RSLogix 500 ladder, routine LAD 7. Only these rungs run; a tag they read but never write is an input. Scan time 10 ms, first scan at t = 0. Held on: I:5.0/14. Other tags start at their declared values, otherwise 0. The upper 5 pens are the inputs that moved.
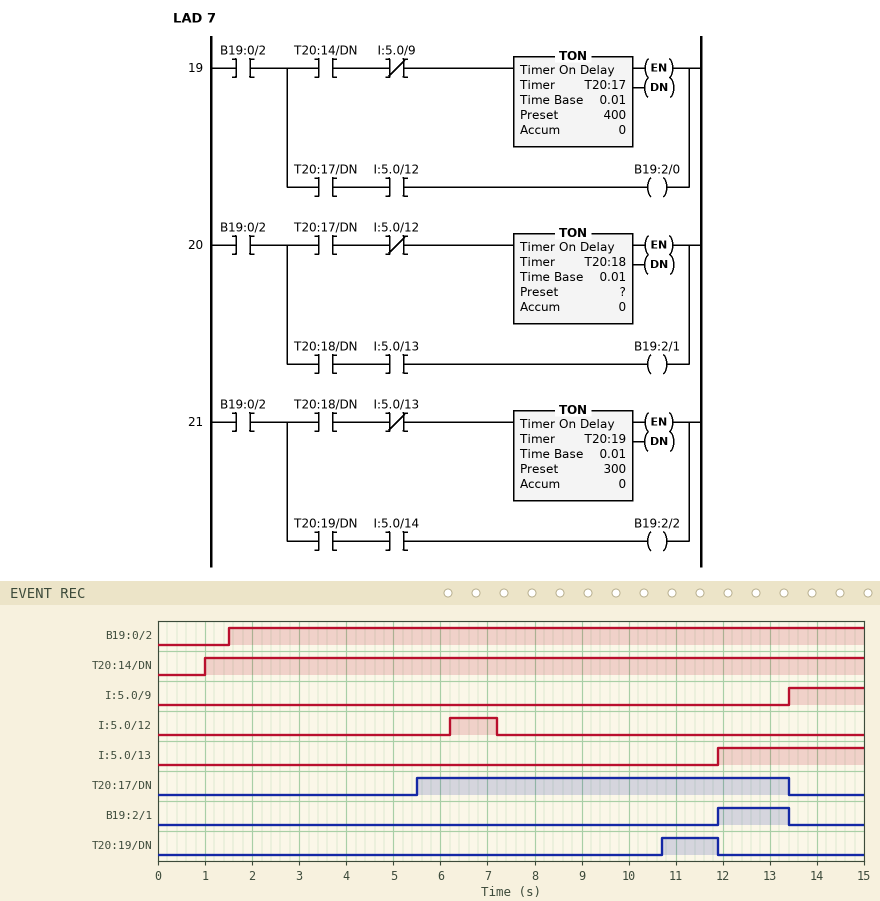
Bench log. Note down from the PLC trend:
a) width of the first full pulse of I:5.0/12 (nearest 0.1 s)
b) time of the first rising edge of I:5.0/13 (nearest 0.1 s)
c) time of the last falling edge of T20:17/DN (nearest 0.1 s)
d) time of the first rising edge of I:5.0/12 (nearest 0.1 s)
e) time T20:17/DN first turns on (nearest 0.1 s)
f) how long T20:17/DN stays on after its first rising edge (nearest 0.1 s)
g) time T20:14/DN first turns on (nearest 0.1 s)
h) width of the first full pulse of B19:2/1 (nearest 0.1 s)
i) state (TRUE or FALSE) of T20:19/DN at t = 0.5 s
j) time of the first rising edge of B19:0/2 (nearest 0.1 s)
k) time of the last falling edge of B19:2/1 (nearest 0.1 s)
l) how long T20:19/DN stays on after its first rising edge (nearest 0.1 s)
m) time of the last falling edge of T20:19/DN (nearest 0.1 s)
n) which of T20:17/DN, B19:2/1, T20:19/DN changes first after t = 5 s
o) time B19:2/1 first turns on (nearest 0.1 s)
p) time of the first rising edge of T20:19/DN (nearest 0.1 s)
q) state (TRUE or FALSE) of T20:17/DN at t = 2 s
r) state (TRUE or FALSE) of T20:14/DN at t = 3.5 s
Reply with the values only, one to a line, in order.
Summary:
1.0 s
11.9 s
13.4 s
6.2 s
5.5 s
7.9 s
1.0 s
1.5 s
FALSE
1.5 s
13.4 s
1.2 s
11.9 s
T20:17/DN
11.9 s
10.7 s
FALSE
TRUE
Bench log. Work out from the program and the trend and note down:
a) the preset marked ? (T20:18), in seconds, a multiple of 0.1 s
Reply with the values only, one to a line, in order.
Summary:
0.5 s
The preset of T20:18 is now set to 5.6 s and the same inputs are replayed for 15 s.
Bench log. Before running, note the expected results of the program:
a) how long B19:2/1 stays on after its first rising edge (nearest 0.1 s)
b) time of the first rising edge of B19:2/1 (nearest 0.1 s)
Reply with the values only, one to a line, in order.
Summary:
0.6 s
12.8 s
